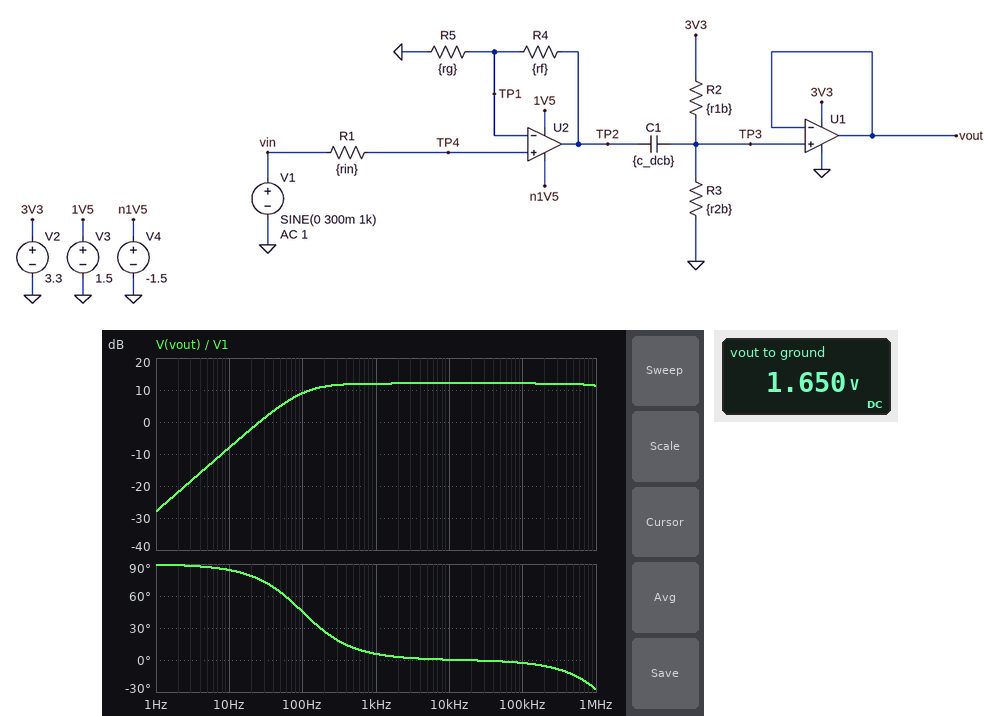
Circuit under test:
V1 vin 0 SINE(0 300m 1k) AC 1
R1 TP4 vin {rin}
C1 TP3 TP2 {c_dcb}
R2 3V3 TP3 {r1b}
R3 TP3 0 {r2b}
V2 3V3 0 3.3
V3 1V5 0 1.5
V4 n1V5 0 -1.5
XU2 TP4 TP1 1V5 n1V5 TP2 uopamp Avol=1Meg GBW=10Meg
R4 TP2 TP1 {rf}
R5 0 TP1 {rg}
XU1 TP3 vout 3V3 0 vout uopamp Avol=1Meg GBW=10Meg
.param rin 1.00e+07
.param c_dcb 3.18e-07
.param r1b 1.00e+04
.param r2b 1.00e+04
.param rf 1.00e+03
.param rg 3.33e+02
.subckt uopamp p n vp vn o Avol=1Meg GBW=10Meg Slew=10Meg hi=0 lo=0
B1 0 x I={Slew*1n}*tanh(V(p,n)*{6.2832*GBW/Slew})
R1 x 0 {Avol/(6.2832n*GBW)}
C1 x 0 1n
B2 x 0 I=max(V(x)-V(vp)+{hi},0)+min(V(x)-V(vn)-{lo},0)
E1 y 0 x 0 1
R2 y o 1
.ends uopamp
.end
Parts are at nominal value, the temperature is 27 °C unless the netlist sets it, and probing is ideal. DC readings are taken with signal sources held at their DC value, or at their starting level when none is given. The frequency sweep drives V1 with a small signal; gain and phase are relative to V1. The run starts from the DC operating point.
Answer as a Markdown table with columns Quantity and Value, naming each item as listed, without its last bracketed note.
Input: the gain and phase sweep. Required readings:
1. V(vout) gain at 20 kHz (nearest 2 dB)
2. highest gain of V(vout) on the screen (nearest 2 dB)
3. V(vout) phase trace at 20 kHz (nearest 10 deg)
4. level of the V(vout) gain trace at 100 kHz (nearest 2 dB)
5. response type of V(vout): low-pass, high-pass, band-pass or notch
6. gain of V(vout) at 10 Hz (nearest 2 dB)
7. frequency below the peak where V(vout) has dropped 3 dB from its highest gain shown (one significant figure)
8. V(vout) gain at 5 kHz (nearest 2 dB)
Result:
| Quantity | Value |
|---|---|
| V(vout) gain at 20 kHz | 12 dB |
| highest gain of V(vout) on the screen | 12 dB |
| V(vout) phase trace at 20 kHz | 0 deg |
| level of the V(vout) gain trace at 100 kHz | 12 dB |
| response type of V(vout): low-pass, high-pass, band-pass or notch | high-pass |
| gain of V(vout) at 10 Hz | -8 dB |
| frequency below the peak where V(vout) has dropped 3 dB from its highest gain shown | 100 Hz |
| V(vout) gain at 5 kHz | 12 dB |
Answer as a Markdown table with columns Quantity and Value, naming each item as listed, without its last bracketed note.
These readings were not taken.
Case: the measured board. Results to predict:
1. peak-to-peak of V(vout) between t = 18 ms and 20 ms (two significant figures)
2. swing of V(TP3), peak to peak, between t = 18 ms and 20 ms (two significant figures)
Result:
| Quantity | Value |
|---|---|
| peak-to-peak of V(vout) between t = 18 ms and 20 ms | 2.4 V |
| swing of V(TP3), peak to peak, between t = 18 ms and 20 ms | 2.4 V |
